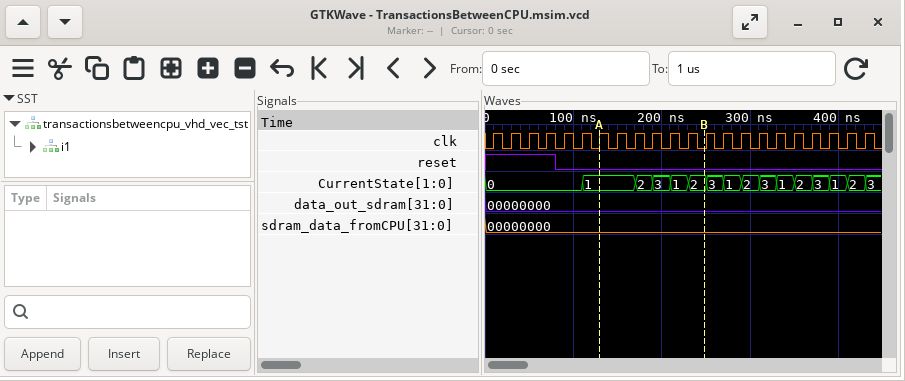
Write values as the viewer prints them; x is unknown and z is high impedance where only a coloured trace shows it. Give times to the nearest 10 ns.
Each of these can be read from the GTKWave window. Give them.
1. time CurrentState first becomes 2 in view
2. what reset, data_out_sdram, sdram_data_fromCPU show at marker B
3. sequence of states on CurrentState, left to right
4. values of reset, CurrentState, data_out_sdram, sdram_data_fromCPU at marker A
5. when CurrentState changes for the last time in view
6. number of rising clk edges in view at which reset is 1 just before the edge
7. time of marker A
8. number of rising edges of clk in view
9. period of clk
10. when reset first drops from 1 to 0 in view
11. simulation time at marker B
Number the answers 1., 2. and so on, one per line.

1. 170 ns
2. reset=0, data_out_sdram=00000000, sdram_data_fromCPU=00000000
3. 0, 1, 2, 3, 1, 2, 3, 1, 2, 3, 1, 2, 3, 1, 2, 3
4. reset=0, CurrentState=1, data_out_sdram=00000000, sdram_data_fromCPU=00000000
5. 430 ns
6. 4
7. 130 ns
8. 22
9. 20 ns
10. 80 ns
11. 250 ns
